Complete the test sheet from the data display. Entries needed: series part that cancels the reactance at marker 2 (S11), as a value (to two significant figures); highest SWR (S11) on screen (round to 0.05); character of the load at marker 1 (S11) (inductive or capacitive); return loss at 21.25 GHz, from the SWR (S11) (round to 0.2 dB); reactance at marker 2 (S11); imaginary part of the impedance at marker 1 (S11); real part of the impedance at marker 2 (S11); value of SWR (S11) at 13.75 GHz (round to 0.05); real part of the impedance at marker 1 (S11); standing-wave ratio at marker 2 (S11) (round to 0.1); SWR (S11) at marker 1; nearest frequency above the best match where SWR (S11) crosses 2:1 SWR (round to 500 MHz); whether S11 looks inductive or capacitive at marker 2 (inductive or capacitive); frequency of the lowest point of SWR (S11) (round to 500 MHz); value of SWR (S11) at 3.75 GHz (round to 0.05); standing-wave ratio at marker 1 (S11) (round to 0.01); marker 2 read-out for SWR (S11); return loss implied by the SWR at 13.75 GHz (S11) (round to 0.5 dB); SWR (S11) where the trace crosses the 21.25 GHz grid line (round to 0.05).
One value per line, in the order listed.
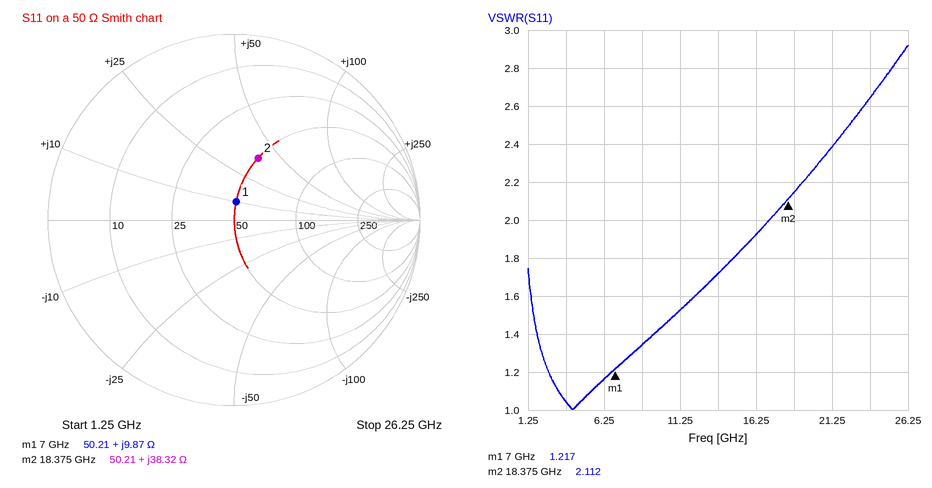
230 fF
2.90
inductive
7.8 dB
+38.32 Ω
+9.87 Ω
50.21 Ω
1.70
50.21 Ω
2.1
1.217
17.0 GHz
inductive
4.0 GHz
1.05
1.22
2.112
11.5 dB
2.40
